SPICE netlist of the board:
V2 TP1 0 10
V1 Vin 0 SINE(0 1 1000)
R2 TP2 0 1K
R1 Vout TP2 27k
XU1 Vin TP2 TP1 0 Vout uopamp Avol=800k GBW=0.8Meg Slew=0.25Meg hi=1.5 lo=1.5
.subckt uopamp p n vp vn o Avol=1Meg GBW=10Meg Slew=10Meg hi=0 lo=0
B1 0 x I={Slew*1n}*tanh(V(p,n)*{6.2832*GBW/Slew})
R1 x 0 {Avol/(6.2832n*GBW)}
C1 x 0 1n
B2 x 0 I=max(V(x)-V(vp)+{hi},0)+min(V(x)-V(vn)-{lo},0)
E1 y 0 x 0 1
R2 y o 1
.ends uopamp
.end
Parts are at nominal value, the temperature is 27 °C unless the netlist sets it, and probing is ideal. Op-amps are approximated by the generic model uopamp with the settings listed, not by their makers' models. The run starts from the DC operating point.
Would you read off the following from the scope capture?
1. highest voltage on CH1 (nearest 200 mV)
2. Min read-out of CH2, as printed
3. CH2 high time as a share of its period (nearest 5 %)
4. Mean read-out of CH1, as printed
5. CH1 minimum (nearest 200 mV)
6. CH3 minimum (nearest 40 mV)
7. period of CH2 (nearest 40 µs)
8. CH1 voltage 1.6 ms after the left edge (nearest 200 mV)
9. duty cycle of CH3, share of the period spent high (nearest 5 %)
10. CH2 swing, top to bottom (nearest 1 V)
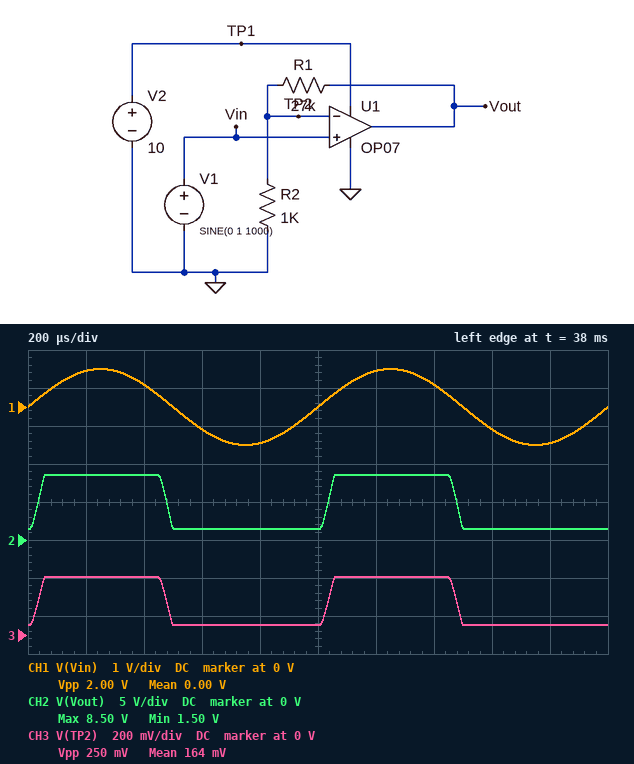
1.0 V
1.50 V
45 %
0.00 V
-1.0 V
40 mV
1.00 ms
-600 mV
45 %
7 V
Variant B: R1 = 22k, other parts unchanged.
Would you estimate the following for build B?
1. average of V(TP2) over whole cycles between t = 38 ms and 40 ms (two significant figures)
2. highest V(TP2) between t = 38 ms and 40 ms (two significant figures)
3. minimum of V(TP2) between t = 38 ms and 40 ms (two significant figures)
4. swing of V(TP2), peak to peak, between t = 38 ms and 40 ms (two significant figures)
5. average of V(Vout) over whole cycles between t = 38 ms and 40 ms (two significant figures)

200 mV
370 mV
65 mV
300 mV
4.5 V
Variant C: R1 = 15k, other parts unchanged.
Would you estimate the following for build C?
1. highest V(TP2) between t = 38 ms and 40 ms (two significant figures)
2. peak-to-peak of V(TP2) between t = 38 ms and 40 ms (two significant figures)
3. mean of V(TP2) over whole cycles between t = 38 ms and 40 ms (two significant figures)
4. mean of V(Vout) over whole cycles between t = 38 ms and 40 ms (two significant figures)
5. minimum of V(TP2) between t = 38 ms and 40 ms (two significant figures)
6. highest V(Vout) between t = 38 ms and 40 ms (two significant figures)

530 mV
440 mV
270 mV
4.3 V
94 mV
8.5 V
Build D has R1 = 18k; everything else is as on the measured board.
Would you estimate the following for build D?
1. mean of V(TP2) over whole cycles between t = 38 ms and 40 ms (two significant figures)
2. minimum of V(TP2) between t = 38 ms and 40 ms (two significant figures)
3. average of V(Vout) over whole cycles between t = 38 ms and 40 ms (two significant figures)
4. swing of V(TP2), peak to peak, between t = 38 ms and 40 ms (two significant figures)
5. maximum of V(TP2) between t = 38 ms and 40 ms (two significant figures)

230 mV
79 mV
4.4 V
370 mV
450 mV
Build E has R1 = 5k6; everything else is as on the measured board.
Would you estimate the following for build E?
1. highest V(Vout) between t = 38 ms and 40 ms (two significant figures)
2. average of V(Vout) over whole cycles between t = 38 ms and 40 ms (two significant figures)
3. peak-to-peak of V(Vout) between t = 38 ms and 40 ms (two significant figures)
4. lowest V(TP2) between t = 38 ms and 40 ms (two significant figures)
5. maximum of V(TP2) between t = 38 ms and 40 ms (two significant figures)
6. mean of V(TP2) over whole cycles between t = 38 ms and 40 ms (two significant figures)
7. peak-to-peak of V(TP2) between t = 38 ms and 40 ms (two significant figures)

6.6 V
2.9 V
5.1 V
230 mV
1.0 V
440 mV
770 mV
